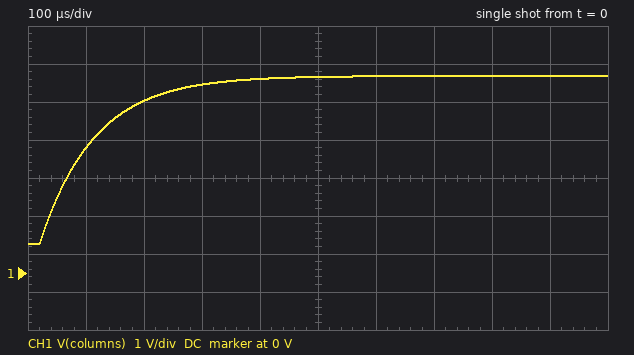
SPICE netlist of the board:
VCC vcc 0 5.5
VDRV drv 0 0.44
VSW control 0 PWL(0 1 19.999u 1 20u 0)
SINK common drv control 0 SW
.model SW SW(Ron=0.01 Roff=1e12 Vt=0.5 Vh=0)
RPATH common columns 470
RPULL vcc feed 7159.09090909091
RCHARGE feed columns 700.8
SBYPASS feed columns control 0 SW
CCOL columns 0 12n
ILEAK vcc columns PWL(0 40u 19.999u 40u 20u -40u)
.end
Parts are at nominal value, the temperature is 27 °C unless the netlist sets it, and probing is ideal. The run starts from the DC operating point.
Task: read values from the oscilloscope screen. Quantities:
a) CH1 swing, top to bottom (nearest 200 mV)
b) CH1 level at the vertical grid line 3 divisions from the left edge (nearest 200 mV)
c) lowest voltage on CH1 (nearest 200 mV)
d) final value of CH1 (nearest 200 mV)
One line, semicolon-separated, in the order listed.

4.4 V; 5.0 V; 800 mV; 5.2 V
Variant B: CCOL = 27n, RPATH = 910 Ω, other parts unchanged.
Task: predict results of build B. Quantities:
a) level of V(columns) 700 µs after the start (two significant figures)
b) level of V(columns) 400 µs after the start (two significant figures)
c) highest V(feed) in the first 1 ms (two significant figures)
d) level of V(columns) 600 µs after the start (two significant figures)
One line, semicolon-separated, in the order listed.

5.0 V; 4.5 V; 5.2 V; 4.9 V
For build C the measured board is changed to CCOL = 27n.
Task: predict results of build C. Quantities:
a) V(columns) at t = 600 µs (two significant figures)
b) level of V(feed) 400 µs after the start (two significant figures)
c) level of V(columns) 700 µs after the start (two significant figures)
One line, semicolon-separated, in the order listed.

4.9 V; 4.5 V; 5.0 V
